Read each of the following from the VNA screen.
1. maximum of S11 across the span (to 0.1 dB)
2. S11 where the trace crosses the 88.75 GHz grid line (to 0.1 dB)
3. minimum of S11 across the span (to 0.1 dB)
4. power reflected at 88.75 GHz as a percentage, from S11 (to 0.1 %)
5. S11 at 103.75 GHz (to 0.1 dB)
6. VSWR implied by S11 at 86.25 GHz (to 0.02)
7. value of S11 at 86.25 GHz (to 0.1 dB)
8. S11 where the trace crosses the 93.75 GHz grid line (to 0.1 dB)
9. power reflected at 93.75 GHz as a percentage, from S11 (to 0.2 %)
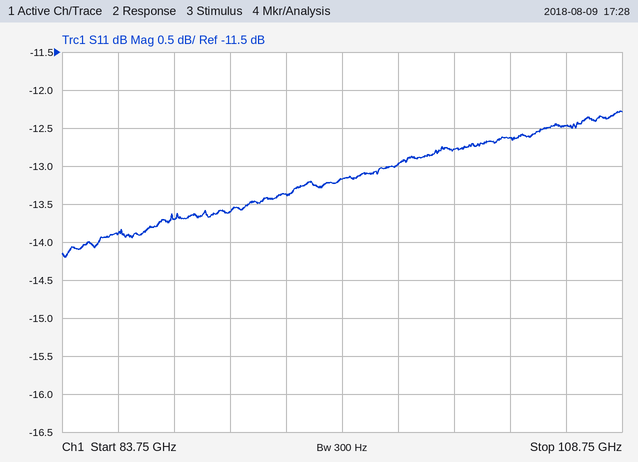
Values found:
-12.3 dB
-13.7 dB
-14.2 dB
4.3 %
-12.6 dB
1.50
-13.9 dB
-13.4 dB
4.6 %
